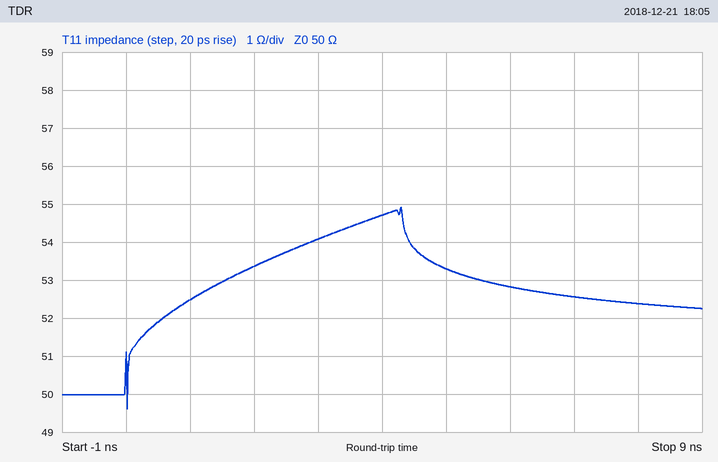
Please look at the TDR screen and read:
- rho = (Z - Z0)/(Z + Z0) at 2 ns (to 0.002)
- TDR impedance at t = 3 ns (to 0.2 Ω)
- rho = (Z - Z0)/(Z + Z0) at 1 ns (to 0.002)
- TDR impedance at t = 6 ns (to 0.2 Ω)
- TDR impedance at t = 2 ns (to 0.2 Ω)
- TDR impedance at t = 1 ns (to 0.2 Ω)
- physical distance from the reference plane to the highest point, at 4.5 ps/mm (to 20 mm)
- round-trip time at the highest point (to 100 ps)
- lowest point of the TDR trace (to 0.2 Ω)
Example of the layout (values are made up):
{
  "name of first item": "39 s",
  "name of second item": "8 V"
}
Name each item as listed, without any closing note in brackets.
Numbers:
{
  "rho = (Z - Z0)/(Z + Z0) at 2 ns": "+0.032",
  "TDR impedance at t = 3 ns": "54.0 Ω",
  "rho = (Z - Z0)/(Z + Z0) at 1 ns": "+0.024",
  "TDR impedance at t = 6 ns": "52.8 Ω",
  "TDR impedance at t = 2 ns": "53.4 Ω",
  "TDR impedance at t = 1 ns": "52.4 Ω",
  "physical distance from the reference plane to the highest point, at 4.5 ps/mm": "480 mm",
  "round-trip time at the highest point": "4.3 ns",
  "lowest point of the TDR trace": "49.6 Ω"
}
